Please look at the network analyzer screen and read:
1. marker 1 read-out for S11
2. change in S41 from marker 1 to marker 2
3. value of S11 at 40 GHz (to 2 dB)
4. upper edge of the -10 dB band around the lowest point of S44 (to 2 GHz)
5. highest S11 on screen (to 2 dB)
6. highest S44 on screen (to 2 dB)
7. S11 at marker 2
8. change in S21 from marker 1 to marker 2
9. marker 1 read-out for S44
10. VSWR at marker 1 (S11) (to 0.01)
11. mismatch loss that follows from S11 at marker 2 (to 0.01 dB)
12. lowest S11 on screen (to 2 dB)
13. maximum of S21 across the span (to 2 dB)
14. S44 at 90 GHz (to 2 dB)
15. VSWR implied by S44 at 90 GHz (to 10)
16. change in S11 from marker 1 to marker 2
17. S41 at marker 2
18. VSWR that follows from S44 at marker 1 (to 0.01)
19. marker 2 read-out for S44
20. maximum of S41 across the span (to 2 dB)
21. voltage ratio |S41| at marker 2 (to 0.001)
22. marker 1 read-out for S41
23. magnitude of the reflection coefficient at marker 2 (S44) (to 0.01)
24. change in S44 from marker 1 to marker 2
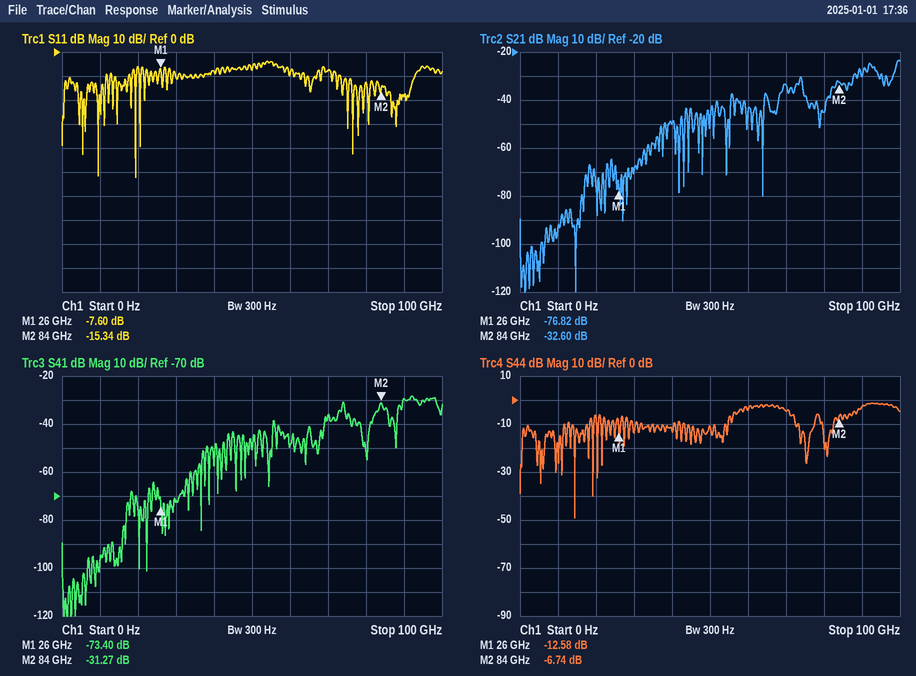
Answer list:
-7.60 dB
42.13 dB
-8 dB
18 GHz
-4 dB
-2 dB
-15.34 dB
44.22 dB
-12.58 dB
2.43
0.13 dB
-52 dB
-24 dB
-2 dB
10
-7.74 dB
-31.27 dB
1.61
-6.74 dB
-28 dB
0.027
-73.40 dB
0.46
5.84 dB
